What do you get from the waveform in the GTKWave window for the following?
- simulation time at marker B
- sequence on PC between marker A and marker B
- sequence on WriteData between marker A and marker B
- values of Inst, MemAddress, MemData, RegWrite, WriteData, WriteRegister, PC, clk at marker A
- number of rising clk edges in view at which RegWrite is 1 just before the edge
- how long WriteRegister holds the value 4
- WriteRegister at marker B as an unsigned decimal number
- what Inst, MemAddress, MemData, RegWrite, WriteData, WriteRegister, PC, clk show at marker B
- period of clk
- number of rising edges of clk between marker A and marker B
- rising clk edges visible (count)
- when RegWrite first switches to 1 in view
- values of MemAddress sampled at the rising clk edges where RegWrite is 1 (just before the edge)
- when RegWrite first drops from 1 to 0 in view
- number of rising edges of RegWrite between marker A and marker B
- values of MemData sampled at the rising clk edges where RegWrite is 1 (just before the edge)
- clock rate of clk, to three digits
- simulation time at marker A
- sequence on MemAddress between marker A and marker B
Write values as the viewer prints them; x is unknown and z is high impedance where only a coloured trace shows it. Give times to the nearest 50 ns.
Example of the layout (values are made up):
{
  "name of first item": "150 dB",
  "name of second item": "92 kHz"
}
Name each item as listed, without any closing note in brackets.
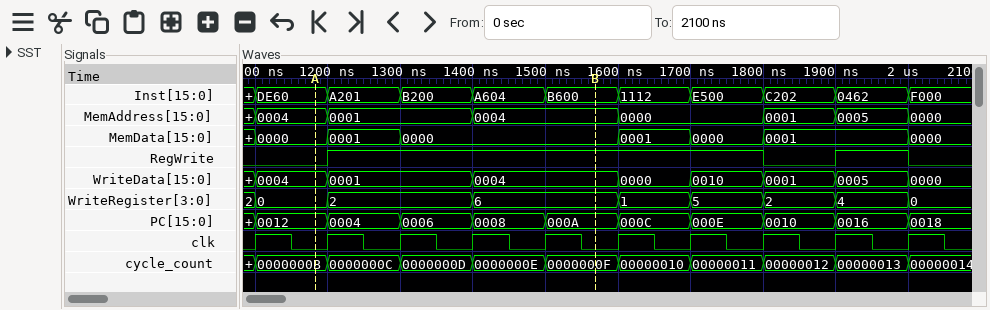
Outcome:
{
  "simulation time at marker B": "1550 ns",
  "sequence on PC between marker A and marker B": "0012, 0004, 0006, 0008, 000A",
  "sequence on WriteData between marker A and marker B": "0004, 0001, 0004",
  "values of Inst, MemAddress, MemData, RegWrite, WriteData, WriteRegister, PC, clk at marker A": "Inst=DE60, MemAddress=0004, MemData=0000, RegWrite=0, WriteData=0004, WriteRegister=0, PC=0012, clk=0",
  "number of rising clk edges in view at which RegWrite is 1 just before the edge": "7",
  "how long WriteRegister holds the value 4": "100 ns",
  "WriteRegister at marker B as an unsigned decimal number": "6",
  "what Inst, MemAddress, MemData, RegWrite, WriteData, WriteRegister, PC, clk show at marker B": "Inst=B600, MemAddress=0004, MemData=0000, RegWrite=1, WriteData=0004, WriteRegister=6, PC=000A, clk=0",
  "period of clk": "100 ns",
  "number of rising edges of clk between marker A and marker B": "4",
  "rising clk edges visible": "10",
  "when RegWrite first switches to 1 in view": "1200 ns",
  "values of MemAddress sampled at the rising clk edges where RegWrite is 1": "0001, 0001, 0004, 0004, 0000, 0000, 0005",
  "when RegWrite first drops from 1 to 0 in view": "1800 ns",
  "number of rising edges of RegWrite between marker A and marker B": "1",
  "values of MemData sampled at the rising clk edges where RegWrite is 1": "0001, 0000, 0000, 0000, 0001, 0000, 0001",
  "clock rate of clk, to three digits": "10.0 MHz",
  "simulation time at marker A": "1200 ns",
  "sequence on MemAddress between marker A and marker B": "0004, 0001, 0004"
}
